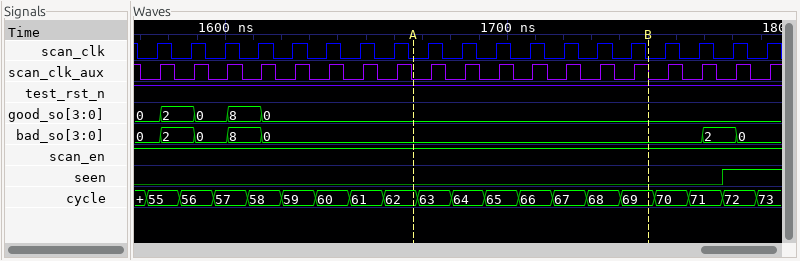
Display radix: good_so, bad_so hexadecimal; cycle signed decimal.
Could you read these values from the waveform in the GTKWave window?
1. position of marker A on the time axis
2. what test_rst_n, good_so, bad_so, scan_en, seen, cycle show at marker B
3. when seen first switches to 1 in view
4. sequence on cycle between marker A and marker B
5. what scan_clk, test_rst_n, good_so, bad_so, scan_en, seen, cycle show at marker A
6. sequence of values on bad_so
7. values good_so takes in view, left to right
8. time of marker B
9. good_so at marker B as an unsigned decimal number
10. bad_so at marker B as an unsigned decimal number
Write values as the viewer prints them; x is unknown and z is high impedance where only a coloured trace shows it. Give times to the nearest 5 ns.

1665 ns
test_rst_n=1, good_so=0, bad_so=0, scan_en=1, seen=0, cycle=69
1775 ns
62, 63, 64, 65, 66, 67, 68, 69
scan_clk=0, test_rst_n=1, good_so=0, bad_so=0, scan_en=1, seen=0, cycle=62
0, 2, 0, 8, 0, 2, 0
0, 2, 0, 8, 0
1750 ns
0
0
